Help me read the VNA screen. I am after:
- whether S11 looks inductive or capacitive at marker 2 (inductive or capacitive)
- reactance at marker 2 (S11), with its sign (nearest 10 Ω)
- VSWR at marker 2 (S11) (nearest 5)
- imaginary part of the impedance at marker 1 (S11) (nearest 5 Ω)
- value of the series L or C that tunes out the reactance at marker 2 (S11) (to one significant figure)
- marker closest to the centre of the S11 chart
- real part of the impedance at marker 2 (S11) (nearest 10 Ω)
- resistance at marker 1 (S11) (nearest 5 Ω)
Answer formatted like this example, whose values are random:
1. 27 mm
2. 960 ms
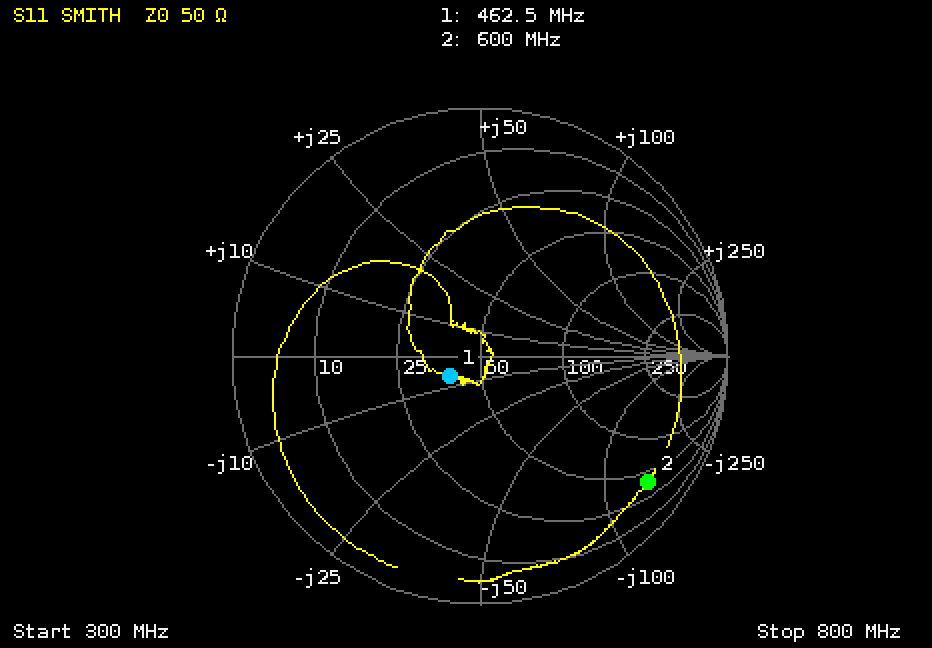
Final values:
1. capacitive
2. -140 Ω
3. 10
4. -5 Ω
5. 40 nH
6. marker 1
7. 40 Ω
8. 40 Ω
